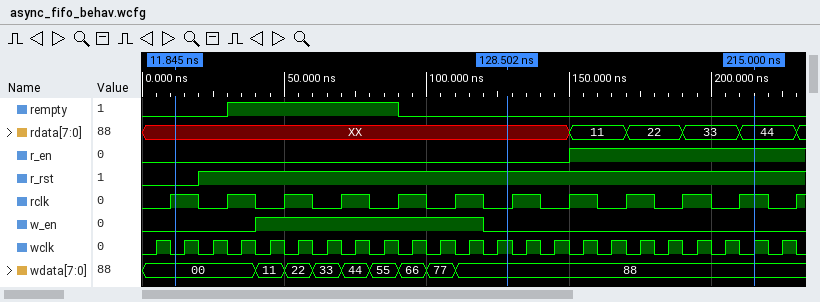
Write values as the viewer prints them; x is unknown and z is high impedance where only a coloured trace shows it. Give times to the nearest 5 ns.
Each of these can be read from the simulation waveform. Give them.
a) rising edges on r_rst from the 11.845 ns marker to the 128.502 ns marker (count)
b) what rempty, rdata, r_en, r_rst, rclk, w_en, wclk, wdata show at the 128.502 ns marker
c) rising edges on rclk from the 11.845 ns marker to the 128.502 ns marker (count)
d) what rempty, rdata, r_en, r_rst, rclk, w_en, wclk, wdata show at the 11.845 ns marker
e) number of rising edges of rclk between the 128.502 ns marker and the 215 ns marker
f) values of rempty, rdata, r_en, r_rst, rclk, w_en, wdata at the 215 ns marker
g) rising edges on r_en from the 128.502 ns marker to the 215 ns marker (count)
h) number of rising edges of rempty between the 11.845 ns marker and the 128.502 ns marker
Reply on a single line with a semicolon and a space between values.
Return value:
1; rempty=0, rdata=XX, r_en=0, r_rst=1, rclk=0, w_en=0, wclk=1, wdata=88; 5; rempty=0, rdata=XX, r_en=0, r_rst=0, rclk=1, w_en=0, wclk=0, wdata=00; 5; rempty=0, rdata=44, r_en=1, r_rst=1, rclk=1, w_en=0, wdata=88; 1; 1
